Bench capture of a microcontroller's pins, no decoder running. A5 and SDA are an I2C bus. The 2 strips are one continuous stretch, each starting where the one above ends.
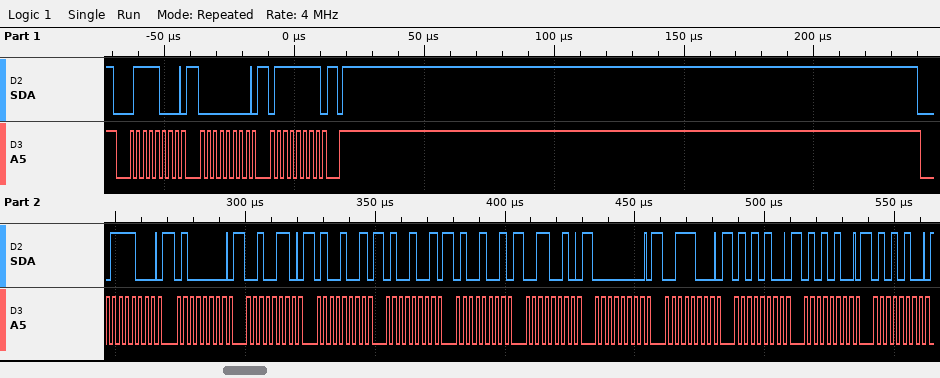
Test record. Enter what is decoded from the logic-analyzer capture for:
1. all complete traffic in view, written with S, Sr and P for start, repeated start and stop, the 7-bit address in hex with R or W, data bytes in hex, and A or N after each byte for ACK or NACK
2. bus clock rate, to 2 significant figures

S 3CW A 00 A 7F A P S 3CW A 40 A 26 A 49 A 49 A 49 A 32 A 00 A 38 A 54 A 54 A 54 A
400 kHz
